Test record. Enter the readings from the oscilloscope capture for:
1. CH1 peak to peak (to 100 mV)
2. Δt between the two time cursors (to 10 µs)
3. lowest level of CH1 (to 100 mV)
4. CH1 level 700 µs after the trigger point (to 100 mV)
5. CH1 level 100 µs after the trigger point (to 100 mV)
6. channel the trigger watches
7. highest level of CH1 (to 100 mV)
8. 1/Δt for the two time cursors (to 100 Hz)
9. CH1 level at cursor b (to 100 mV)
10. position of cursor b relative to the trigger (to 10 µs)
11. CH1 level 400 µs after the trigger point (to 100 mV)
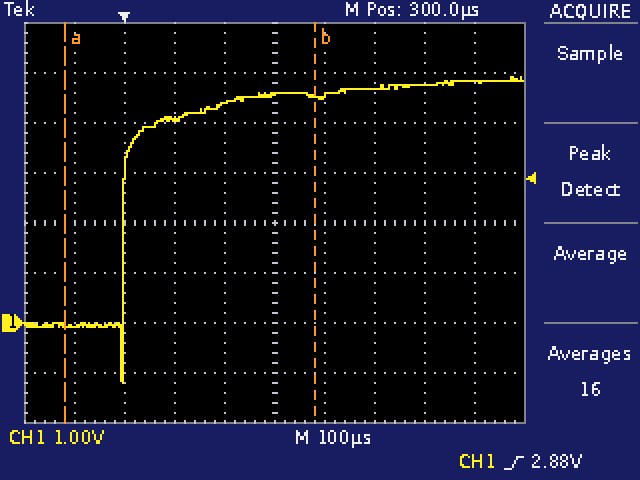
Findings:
6.1 V
500 µs
-1.2 V
4.8 V
4.1 V
CH1
4.9 V
2.0 kHz
4.5 V
+380 µs
4.5 V
